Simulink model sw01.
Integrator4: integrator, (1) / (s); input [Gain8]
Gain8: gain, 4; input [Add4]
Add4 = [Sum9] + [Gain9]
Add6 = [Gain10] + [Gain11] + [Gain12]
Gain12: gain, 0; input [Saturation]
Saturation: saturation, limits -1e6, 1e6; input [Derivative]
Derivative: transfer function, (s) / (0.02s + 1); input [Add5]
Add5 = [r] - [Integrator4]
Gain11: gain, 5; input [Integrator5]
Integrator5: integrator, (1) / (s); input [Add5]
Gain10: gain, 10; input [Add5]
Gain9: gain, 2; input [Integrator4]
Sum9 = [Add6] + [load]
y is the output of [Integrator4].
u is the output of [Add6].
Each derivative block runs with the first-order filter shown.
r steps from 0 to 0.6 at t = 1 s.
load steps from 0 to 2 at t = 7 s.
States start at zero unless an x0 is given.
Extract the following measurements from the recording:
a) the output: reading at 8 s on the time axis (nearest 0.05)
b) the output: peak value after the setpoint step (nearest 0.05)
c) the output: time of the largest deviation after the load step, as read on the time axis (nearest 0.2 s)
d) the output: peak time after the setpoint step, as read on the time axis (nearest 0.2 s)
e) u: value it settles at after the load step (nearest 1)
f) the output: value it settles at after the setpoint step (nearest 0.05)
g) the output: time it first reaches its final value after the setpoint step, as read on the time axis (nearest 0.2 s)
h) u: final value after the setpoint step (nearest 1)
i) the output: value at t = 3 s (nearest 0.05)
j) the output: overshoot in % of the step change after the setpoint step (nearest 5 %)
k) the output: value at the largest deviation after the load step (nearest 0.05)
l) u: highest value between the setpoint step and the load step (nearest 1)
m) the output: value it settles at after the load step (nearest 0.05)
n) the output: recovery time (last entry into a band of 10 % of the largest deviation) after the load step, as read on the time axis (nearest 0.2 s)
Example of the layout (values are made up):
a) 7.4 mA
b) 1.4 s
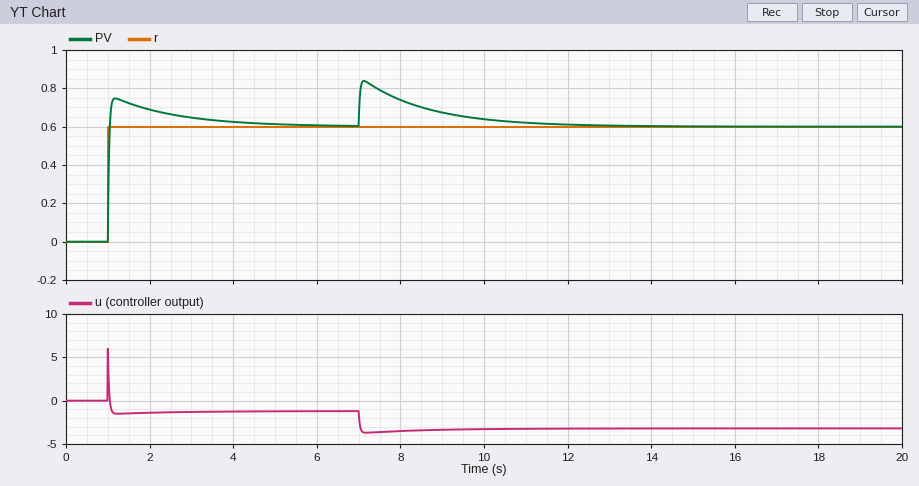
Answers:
a) 0.75
b) 0.75
c) 7.2 s
d) 1.2 s
e) -3
f) 0.60
g) 1.0 s
h) -1
i) 0.65
j) 25 %
k) 0.85
l) 6
m) 0.60
n) 10.8 s
